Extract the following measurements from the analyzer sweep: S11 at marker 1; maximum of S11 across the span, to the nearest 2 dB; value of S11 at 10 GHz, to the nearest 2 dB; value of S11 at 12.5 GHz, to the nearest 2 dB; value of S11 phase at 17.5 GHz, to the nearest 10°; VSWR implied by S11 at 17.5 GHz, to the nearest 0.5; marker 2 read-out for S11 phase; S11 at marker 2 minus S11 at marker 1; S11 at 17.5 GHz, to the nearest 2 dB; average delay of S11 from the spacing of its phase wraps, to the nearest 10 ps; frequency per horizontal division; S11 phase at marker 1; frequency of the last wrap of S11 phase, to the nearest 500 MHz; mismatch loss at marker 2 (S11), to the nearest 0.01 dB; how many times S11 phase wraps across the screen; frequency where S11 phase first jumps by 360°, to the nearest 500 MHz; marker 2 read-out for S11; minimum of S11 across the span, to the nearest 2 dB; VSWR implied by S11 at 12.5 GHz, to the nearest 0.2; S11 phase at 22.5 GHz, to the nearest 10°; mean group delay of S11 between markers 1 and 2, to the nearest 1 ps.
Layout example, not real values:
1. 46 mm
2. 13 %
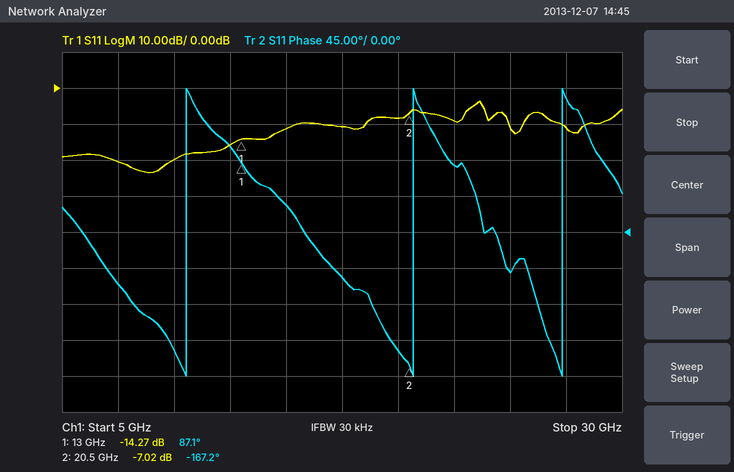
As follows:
1. -14.27 dB
2. -4 dB
3. -20 dB
4. -16 dB
5. -60°
6. 2.0
7. -167.2°
8. 7.25 dB
9. -10 dB
10. 120 ps
11. 2.5 GHz
12. 87.1°
13. 27.5 GHz
14. 0.96 dB
15. 3
16. 10.5 GHz
17. -7.02 dB
18. -24 dB
19. 1.4
20. 80°
21. 94 ps
